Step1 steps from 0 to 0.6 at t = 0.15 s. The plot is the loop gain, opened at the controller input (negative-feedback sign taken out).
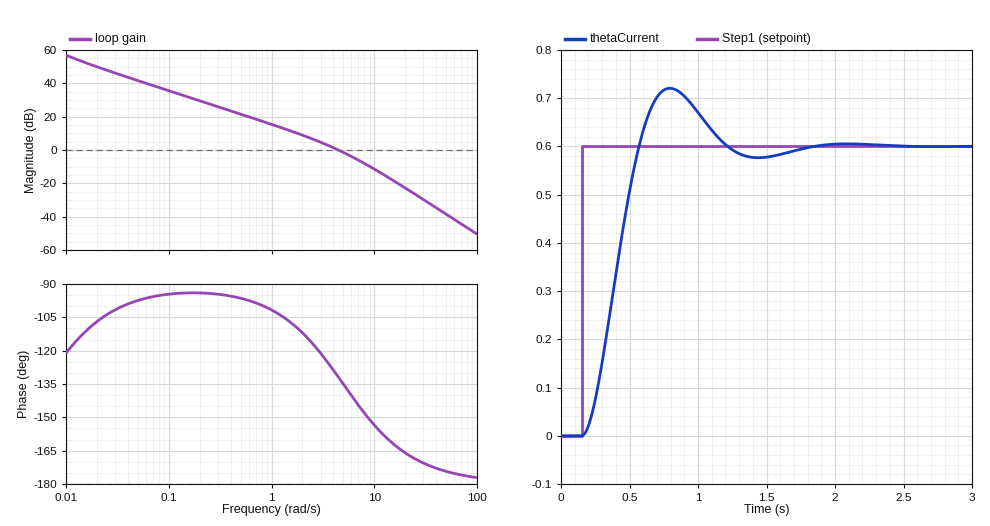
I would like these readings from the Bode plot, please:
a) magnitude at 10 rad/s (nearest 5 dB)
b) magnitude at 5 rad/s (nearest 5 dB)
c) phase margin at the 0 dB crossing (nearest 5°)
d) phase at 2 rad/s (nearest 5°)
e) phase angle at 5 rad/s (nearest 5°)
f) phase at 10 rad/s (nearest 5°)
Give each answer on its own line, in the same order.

-10 dB
0 dB
50°
-110°
-135°
-155°
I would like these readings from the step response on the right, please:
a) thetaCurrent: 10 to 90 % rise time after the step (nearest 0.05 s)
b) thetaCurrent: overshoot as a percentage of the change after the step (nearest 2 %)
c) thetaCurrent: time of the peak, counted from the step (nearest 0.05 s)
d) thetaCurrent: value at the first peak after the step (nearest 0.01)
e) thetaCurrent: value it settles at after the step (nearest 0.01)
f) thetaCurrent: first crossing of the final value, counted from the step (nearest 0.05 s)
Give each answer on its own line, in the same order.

0.30 s
20 %
0.65 s
0.72
0.60
0.40 s
